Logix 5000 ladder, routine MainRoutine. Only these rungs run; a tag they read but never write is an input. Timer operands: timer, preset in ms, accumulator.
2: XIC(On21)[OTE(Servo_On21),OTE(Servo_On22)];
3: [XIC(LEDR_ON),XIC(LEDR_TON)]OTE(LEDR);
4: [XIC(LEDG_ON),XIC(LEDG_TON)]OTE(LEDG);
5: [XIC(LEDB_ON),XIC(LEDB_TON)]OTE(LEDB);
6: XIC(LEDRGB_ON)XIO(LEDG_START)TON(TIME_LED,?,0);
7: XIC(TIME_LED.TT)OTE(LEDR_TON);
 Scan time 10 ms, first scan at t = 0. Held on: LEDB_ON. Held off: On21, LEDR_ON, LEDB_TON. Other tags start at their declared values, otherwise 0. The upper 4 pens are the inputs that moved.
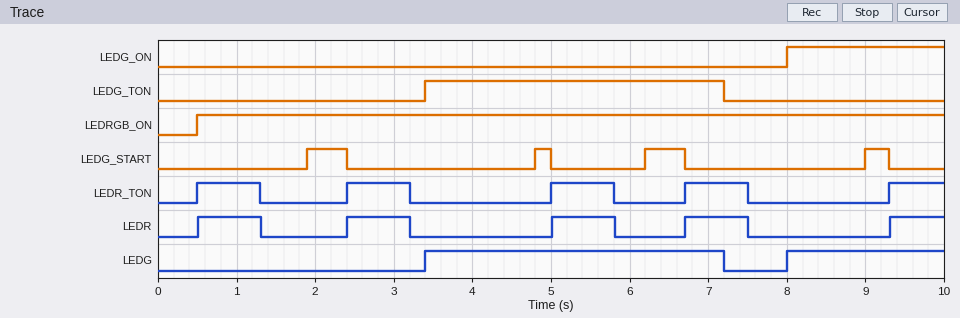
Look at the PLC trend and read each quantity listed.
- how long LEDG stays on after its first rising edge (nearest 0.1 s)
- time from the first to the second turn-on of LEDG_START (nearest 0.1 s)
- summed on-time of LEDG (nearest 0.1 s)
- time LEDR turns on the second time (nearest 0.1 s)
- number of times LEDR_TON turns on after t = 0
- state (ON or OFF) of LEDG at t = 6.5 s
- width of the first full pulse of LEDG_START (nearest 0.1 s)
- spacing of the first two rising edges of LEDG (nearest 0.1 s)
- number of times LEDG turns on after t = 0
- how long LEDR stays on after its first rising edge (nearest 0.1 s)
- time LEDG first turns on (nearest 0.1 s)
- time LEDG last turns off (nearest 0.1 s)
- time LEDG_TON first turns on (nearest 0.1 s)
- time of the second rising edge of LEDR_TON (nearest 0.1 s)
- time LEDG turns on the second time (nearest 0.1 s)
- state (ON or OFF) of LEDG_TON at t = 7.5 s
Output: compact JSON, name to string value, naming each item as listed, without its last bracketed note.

{"how long LEDG stays on after its first rising edge": "3.8 s", "time from the first to the second turn-on of LEDG_START": "2.9 s", "summed on-time of LEDG": "5.8 s", "time LEDR turns on the second time": "2.4 s", "number of times LEDR_TON turns on after t = 0": "5", "state (ON or OFF) of LEDG at t = 6.5 s": "ON", "width of the first full pulse of LEDG_START": "0.5 s", "spacing of the first two rising edges of LEDG": "4.6 s", "number of times LEDG turns on after t = 0": "2", "how long LEDR stays on after its first rising edge": "0.8 s", "time LEDG first turns on": "3.4 s", "time LEDG last turns off": "7.2 s", "time LEDG_TON first turns on": "3.4 s", "time of the second rising edge of LEDR_TON": "2.4 s", "time LEDG turns on the second time": "8.0 s", "state (ON or OFF) of LEDG_TON at t = 7.5 s": "OFF"}
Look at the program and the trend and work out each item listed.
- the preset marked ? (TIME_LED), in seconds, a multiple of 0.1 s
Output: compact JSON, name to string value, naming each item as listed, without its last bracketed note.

{"the preset marked ? (TIME_LED), in seconds, a multiple of 0.1 s": "0.8 s"}
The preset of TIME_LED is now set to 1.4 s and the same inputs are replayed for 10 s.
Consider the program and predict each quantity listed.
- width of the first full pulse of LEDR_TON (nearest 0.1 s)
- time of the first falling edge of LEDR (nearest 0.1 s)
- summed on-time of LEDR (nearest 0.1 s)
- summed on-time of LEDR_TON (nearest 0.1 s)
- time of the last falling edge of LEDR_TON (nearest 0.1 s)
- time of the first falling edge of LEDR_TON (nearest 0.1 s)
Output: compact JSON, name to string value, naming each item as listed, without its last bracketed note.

{"width of the first full pulse of LEDR_TON": "1.4 s", "time of the first falling edge of LEDR": "1.9 s", "summed on-time of LEDR": "6.1 s", "summed on-time of LEDR_TON": "6.1 s", "time of the last falling edge of LEDR_TON": "8.1 s", "time of the first falling edge of LEDR_TON": "1.9 s"}
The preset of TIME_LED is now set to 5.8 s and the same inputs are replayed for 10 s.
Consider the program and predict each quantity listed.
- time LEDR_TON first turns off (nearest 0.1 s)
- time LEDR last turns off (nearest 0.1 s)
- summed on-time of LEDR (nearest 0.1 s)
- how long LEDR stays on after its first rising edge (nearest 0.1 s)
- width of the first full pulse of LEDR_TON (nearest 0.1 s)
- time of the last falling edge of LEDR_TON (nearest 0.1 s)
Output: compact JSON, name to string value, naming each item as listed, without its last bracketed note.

{"time LEDR_TON first turns off": "1.9 s", "time LEDR last turns off": "9.0 s", "summed on-time of LEDR": "8.0 s", "how long LEDR stays on after its first rising edge": "1.4 s", "width of the first full pulse of LEDR_TON": "1.4 s", "time of the last falling edge of LEDR_TON": "9.0 s"}
